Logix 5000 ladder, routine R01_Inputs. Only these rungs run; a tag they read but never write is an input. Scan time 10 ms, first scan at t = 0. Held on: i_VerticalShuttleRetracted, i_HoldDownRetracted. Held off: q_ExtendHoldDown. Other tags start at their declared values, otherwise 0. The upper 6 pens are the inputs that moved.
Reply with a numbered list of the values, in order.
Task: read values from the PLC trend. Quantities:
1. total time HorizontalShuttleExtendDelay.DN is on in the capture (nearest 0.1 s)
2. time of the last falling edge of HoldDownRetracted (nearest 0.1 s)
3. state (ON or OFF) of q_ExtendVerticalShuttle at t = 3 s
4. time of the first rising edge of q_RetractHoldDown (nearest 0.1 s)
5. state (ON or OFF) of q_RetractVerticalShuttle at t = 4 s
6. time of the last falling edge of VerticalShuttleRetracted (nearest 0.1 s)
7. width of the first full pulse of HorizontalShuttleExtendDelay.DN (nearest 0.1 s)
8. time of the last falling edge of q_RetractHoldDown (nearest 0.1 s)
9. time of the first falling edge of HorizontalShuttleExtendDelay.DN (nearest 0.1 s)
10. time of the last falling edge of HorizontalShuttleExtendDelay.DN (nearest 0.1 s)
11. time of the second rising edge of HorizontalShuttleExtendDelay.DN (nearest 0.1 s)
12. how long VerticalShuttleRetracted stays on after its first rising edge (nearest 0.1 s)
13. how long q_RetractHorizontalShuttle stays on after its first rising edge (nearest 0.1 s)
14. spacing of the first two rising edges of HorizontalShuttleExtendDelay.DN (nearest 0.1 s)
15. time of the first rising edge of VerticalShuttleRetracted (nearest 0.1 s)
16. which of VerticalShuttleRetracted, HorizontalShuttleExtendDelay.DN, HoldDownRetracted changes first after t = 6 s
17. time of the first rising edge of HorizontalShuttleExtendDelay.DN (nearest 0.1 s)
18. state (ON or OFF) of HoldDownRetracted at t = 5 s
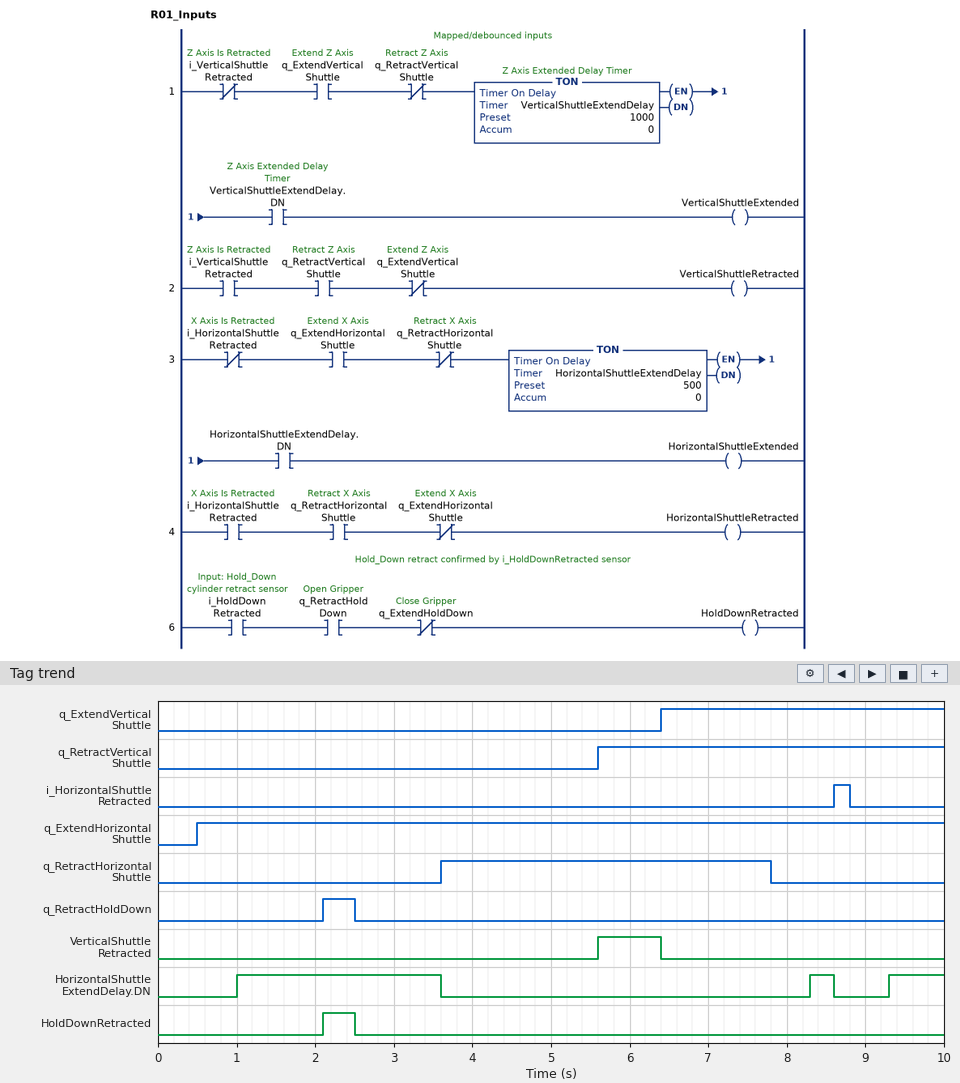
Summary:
1. 3.6 s
2. 2.5 s
3. OFF
4. 2.1 s
5. OFF
6. 6.4 s
7. 2.6 s
8. 2.5 s
9. 3.6 s
10. 8.6 s
11. 8.3 s
12. 0.8 s
13. 4.2 s
14. 7.3 s
15. 5.6 s
16. VerticalShuttleRetracted
17. 1.0 s
18. OFF
